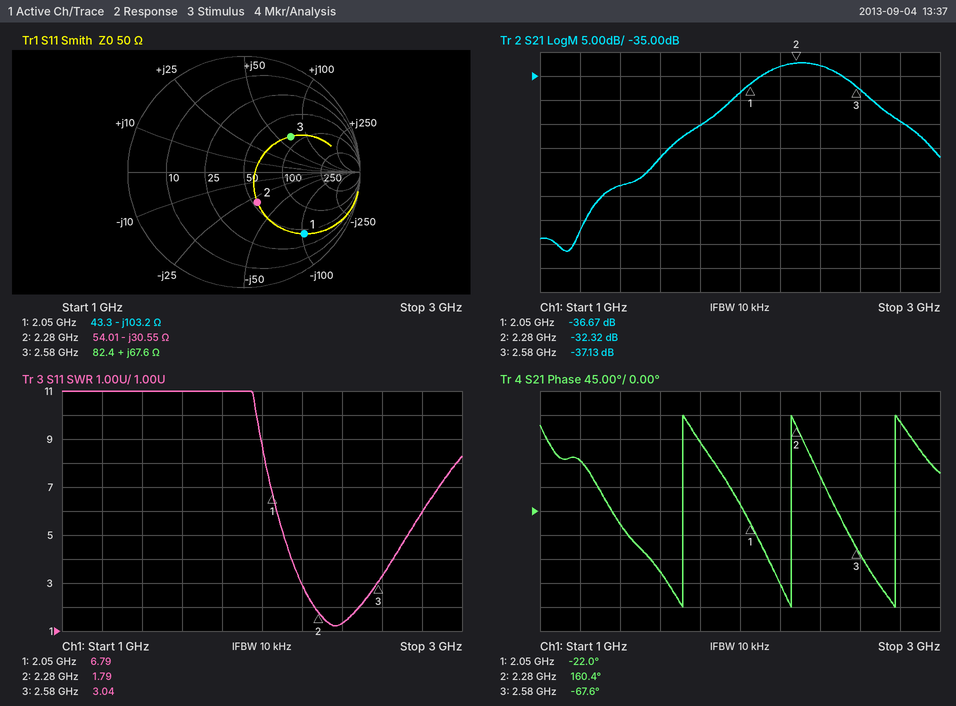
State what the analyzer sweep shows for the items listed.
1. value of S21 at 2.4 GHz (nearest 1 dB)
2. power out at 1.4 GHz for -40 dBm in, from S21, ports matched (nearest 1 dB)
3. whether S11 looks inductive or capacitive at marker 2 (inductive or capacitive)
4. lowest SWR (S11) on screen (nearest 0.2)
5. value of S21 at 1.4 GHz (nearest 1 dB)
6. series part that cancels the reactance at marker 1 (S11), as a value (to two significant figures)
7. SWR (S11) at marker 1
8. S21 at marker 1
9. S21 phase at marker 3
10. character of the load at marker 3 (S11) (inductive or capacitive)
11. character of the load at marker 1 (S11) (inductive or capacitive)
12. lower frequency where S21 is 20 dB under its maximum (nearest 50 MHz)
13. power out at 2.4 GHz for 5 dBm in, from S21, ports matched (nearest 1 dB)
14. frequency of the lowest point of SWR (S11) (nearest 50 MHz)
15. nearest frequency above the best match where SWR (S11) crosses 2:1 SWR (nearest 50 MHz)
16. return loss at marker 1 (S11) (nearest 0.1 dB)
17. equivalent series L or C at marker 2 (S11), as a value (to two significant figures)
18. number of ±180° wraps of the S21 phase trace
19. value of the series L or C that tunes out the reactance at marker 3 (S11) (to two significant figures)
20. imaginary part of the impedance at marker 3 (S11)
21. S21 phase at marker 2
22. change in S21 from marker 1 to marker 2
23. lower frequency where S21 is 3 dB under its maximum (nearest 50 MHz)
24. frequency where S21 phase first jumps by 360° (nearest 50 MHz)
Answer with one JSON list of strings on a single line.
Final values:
["-33 dB", "-98 dBm", "capacitive", "1.2", "-58 dB", "8.0 nH", "6.79", "-36.67 dB", "-67.6°", "inductive", "capacitive", "1.60 GHz", "-28 dBm", "2.35 GHz", "2.50 GHz", "2.6 dB", "2.3 pF", "3", "910 fF", "+67.6 Ω", "160.4°", "4.35 dB", "2.10 GHz", "1.70 GHz"]
